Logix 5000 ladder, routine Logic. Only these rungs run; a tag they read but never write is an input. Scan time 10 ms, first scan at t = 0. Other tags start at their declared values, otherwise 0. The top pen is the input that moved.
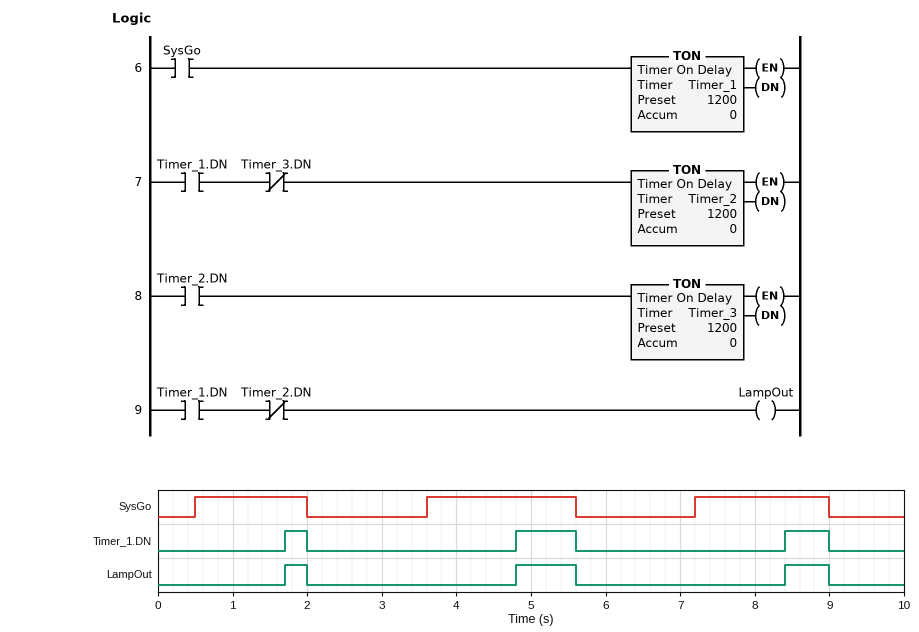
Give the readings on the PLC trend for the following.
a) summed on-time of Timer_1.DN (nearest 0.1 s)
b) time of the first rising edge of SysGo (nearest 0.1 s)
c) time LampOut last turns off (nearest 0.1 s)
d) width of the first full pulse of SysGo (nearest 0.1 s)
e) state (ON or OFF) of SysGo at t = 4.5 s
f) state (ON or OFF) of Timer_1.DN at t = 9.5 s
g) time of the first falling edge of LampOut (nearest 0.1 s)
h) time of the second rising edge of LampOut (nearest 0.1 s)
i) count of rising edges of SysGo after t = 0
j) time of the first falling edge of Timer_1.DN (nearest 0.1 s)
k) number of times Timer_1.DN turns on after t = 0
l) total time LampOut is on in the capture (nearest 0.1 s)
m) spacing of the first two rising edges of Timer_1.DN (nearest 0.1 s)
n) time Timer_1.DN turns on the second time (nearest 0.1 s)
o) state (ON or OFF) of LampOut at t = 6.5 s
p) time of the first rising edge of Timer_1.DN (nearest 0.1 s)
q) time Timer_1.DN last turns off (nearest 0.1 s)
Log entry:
1.7 s
0.5 s
9.0 s
1.5 s
ON
OFF
2.0 s
4.8 s
3
2.0 s
3
1.7 s
3.1 s
4.8 s
OFF
1.7 s
9.0 s
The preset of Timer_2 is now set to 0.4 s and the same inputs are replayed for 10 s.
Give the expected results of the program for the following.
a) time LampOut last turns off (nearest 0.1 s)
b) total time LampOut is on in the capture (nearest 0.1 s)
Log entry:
8.8 s
1.1 s
